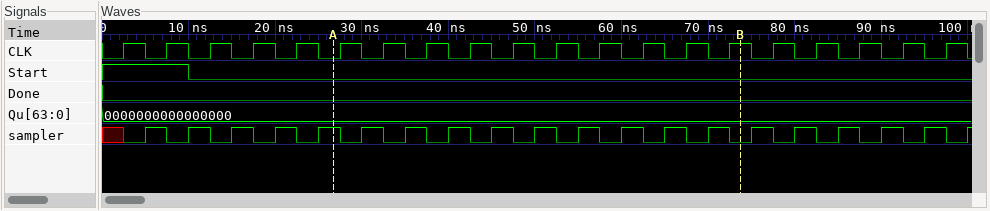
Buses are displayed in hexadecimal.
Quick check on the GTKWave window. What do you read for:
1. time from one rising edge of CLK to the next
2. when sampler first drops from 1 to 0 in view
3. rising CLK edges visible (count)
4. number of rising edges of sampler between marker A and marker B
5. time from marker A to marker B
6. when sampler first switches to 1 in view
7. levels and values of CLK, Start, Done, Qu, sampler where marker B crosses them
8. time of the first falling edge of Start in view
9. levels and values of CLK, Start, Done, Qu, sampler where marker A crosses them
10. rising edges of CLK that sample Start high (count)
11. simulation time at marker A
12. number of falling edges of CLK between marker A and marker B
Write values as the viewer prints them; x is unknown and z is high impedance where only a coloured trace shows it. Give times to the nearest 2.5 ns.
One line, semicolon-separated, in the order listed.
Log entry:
5 ns; 7.5 ns; 20; 9; 47.5 ns; 5 ns; CLK=1, Start=0, Done=0, Qu=0000000000000000, sampler=0; 10 ns; CLK=0, Start=0, Done=0, Qu=0000000000000000, sampler=1; 2; 27.5 ns; 9
